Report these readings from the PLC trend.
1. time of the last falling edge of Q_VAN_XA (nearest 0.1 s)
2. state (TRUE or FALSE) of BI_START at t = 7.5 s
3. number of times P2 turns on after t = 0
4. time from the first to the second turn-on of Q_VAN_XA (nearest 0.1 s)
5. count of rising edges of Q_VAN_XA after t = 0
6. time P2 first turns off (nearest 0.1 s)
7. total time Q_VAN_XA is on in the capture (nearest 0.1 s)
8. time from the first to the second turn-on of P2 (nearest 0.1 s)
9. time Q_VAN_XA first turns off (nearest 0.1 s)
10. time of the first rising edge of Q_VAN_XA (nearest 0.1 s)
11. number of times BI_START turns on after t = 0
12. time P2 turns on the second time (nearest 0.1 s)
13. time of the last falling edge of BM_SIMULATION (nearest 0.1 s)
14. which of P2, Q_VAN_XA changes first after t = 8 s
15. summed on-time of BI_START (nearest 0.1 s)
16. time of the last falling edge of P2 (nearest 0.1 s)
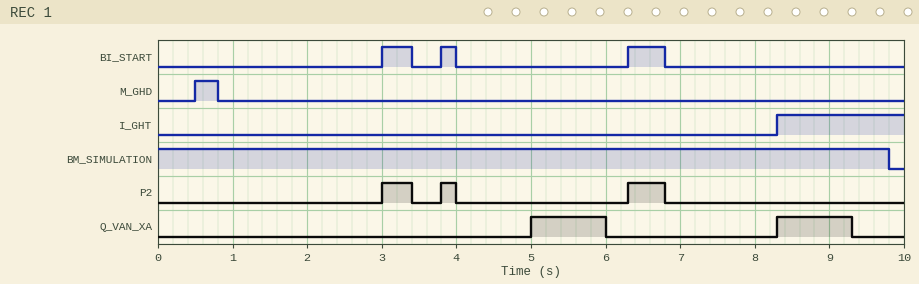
9.3 s
FALSE
3
3.3 s
2
3.4 s
2.0 s
0.8 s
6.0 s
5.0 s
3
3.8 s
9.8 s
Q_VAN_XA
1.1 s
6.8 s
